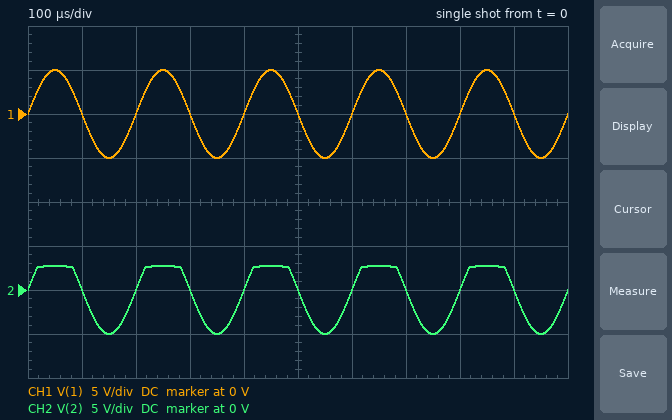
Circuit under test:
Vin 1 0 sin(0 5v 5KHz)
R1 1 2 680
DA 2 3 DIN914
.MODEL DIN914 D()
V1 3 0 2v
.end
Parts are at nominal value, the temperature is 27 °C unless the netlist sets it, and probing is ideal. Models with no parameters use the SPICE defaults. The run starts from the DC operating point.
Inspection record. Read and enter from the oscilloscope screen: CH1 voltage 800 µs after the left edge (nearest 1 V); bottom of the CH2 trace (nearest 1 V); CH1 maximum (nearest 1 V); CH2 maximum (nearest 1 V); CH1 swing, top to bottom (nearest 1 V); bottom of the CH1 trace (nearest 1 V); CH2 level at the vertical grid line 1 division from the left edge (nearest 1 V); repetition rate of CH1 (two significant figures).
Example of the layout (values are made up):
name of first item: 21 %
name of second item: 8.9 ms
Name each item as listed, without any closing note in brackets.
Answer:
CH1 voltage 800 µs after the left edge: 0 V
bottom of the CH2 trace: -5 V
CH1 maximum: 5 V
CH2 maximum: 3 V
CH1 swing, top to bottom: 10 V
bottom of the CH1 trace: -5 V
CH2 level at the vertical grid line 1 division from the left edge: 0 V
repetition rate of CH1: 5.0 kHz
